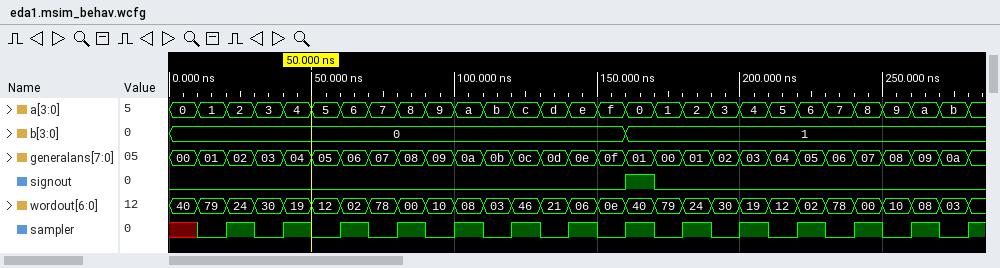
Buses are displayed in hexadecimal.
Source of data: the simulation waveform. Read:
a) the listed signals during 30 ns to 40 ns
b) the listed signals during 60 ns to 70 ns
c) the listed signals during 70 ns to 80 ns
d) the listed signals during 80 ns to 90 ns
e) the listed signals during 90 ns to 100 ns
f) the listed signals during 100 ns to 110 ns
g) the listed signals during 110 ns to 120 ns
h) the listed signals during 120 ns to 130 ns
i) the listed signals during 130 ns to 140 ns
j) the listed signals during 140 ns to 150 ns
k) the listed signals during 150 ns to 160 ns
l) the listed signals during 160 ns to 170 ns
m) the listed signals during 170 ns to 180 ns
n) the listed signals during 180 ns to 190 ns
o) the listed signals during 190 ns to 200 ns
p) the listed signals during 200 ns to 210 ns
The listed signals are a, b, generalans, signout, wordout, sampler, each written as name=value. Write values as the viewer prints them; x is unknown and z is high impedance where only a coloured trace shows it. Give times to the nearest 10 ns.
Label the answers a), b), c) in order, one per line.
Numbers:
a) a=3, b=0, generalans=03, signout=0, wordout=30, sampler=0
b) a=6, b=0, generalans=06, signout=0, wordout=02, sampler=1
c) a=7, b=0, generalans=07, signout=0, wordout=78, sampler=0
d) a=8, b=0, generalans=08, signout=0, wordout=00, sampler=1
e) a=9, b=0, generalans=09, signout=0, wordout=10, sampler=0
f) a=a, b=0, generalans=0a, signout=0, wordout=08, sampler=1
g) a=b, b=0, generalans=0b, signout=0, wordout=03, sampler=0
h) a=c, b=0, generalans=0c, signout=0, wordout=46, sampler=1
i) a=d, b=0, generalans=0d, signout=0, wordout=21, sampler=0
j) a=e, b=0, generalans=0e, signout=0, wordout=06, sampler=1
k) a=f, b=0, generalans=0f, signout=0, wordout=0e, sampler=0
l) a=0, b=1, generalans=01, signout=1, wordout=40, sampler=1
m) a=1, b=1, generalans=00, signout=0, wordout=79, sampler=0
n) a=2, b=1, generalans=01, signout=0, wordout=24, sampler=1
o) a=3, b=1, generalans=02, signout=0, wordout=30, sampler=0
p) a=4, b=1, generalans=03, signout=0, wordout=19, sampler=1
